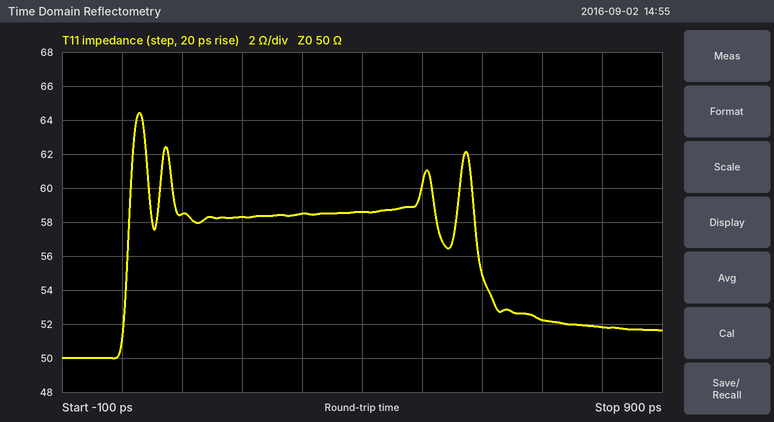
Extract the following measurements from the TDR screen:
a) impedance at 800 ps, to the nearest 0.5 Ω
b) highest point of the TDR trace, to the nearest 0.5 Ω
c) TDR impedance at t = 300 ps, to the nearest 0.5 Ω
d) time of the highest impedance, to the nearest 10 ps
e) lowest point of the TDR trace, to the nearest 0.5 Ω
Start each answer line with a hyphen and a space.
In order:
- 52.0 Ω
- 64.5 Ω
- 58.5 Ω
- 30 ps
- 50.0 Ω
